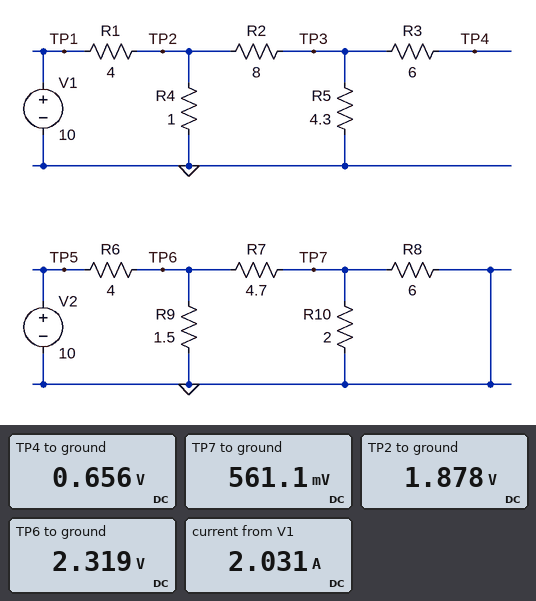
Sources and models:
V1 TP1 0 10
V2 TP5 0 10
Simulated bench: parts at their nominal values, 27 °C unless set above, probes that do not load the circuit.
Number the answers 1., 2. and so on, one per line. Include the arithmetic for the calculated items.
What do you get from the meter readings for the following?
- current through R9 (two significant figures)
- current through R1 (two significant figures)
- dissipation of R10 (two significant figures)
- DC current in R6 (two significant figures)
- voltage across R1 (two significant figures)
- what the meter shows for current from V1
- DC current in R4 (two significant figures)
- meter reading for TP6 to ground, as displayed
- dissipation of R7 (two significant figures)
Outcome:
1. (2.319 V) / 1.5 Ω = 1.5 A
2. (10 V - 1.878 V) / 4 Ω = 2.0 A
3. (561.1 mV)^2 / 2 Ω = 160 mW
4. (10 V - 2.319 V) / 4 Ω = 1.9 A
5. 10 V - 1.878 V = 8.1 V
6. 2.031 A
7. (1.878 V) / 1 Ω = 1.9 A
8. 2.319 V
9. (2.319 V - 561.1 mV)^2 / 4.7 Ω = 660 mW
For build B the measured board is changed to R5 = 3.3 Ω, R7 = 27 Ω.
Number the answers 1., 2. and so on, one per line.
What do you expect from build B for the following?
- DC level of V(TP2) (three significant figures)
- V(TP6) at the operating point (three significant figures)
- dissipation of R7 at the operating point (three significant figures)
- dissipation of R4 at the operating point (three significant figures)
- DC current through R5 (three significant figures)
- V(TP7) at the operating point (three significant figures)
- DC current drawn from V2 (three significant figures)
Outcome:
1. 1.87 V
2. 2.63 V
3. 229 mW
4. 3.49 W
5. 165 mA
6. 138 mV
7. 1.84 A
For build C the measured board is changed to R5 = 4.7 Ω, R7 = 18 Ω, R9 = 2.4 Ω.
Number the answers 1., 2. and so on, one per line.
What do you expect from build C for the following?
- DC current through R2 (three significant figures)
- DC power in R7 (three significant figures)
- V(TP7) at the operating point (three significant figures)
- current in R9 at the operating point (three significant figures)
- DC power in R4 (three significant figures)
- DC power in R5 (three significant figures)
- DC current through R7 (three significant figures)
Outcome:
1. 148 mA
2. 574 mW
3. 268 mV
4. 1.45 A
5. 3.54 W
6. 103 mW
7. 179 mA
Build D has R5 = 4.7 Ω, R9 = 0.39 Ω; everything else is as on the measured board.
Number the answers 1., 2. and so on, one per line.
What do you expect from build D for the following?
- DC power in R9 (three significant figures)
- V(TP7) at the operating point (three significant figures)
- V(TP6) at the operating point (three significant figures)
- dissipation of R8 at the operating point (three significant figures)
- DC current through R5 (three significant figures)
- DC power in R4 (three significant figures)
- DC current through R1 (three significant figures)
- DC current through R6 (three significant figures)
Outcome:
1. 1.81 W
2. 203 mV
3. 840 mV
4. 6.89 mW
5. 148 mA
6. 3.54 W
7. 2.03 A
8. 2.29 A
